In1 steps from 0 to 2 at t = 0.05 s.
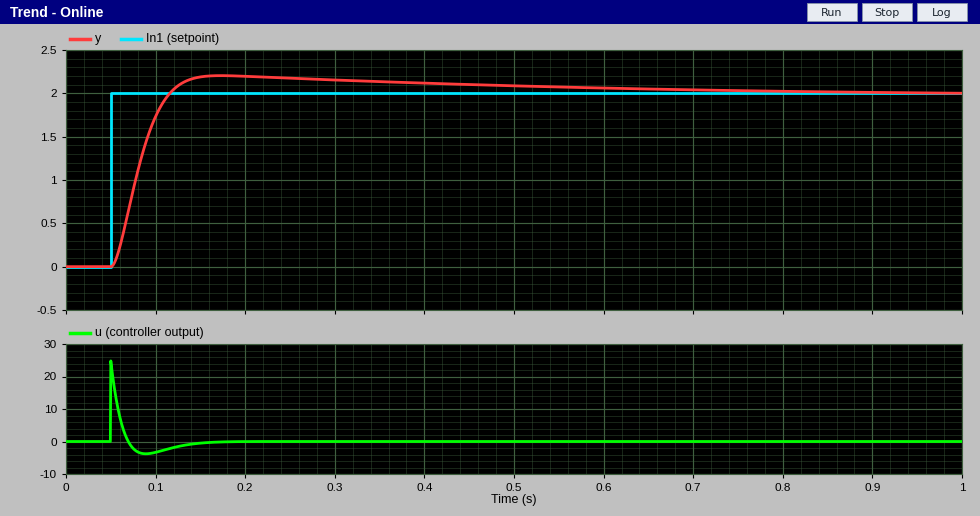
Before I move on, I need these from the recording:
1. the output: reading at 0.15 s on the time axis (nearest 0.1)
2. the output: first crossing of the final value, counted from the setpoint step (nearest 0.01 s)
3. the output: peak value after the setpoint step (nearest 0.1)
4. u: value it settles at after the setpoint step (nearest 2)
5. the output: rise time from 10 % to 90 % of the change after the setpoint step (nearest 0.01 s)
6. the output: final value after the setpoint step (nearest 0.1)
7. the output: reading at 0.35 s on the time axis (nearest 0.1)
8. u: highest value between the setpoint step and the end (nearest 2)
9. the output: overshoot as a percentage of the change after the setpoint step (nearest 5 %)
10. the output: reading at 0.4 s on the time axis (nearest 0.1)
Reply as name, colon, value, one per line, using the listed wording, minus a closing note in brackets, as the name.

the output: reading at 0.15 s on the time axis: 2.2
the output: first crossing of the final value, counted from the setpoint step: 0.07 s
the output: peak value after the setpoint step: 2.2
u: value it settles at after the setpoint step: 0
the output: rise time from 10 % to 90 % of the change after the setpoint step: 0.04 s
the output: final value after the setpoint step: 2.0
the output: reading at 0.35 s on the time axis: 2.1
u: highest value between the setpoint step and the end: 24
the output: overshoot as a percentage of the change after the setpoint step: 10 %
the output: reading at 0.4 s on the time axis: 2.1
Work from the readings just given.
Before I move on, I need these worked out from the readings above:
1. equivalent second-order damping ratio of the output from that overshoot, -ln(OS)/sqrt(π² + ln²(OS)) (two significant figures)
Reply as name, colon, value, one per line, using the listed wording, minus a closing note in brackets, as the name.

equivalent second-order damping ratio of the output from that overshoot, -ln(OS)/sqrt(π² + ln²(OS)): 0.59
